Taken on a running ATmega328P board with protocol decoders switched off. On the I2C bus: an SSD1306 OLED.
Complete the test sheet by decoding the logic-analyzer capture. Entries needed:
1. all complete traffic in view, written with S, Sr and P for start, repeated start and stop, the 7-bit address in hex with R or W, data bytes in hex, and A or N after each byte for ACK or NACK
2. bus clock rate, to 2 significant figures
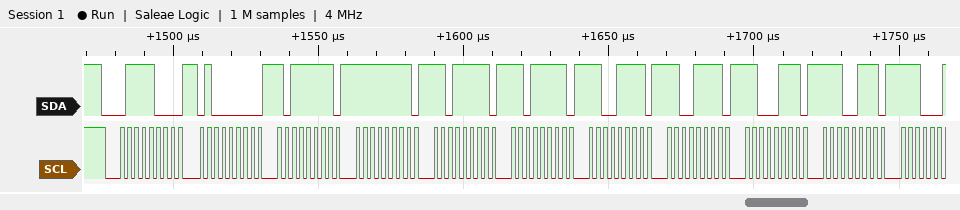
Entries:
S 3CW A 40 A BF A FF A DF A DF A CF A CF A C7 A E7 A
400 kHz
